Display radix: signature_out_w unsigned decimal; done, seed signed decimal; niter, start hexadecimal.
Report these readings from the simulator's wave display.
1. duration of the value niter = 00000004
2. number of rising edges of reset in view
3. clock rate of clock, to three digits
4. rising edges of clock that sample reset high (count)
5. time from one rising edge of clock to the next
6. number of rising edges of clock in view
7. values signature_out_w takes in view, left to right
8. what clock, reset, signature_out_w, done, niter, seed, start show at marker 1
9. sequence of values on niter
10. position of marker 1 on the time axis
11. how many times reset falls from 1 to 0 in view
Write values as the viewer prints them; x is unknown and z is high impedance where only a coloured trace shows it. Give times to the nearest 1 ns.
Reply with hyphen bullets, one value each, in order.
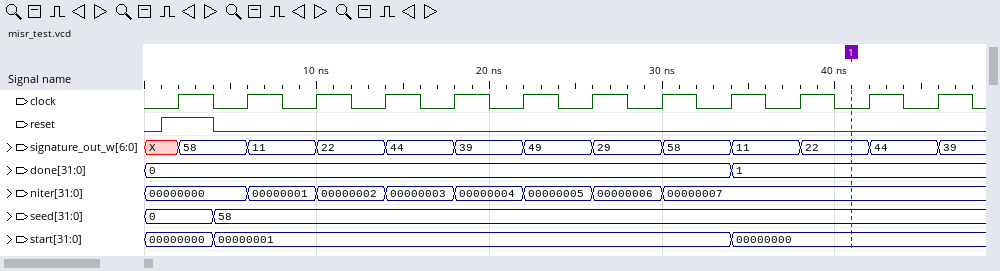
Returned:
- 4 ns
- 1
- 250 MHz
- 1
- 4 ns
- 12
- X, 58, 11, 22, 44, 39, 49, 29, 58, 11, 22, 44, 39
- clock=0, reset=0, signature_out_w=22, done=1, niter=00000007, seed=58, start=00000000
- 00000000, 00000001, 00000002, 00000003, 00000004, 00000005, 00000006, 00000007
- 41 ns
- 1
